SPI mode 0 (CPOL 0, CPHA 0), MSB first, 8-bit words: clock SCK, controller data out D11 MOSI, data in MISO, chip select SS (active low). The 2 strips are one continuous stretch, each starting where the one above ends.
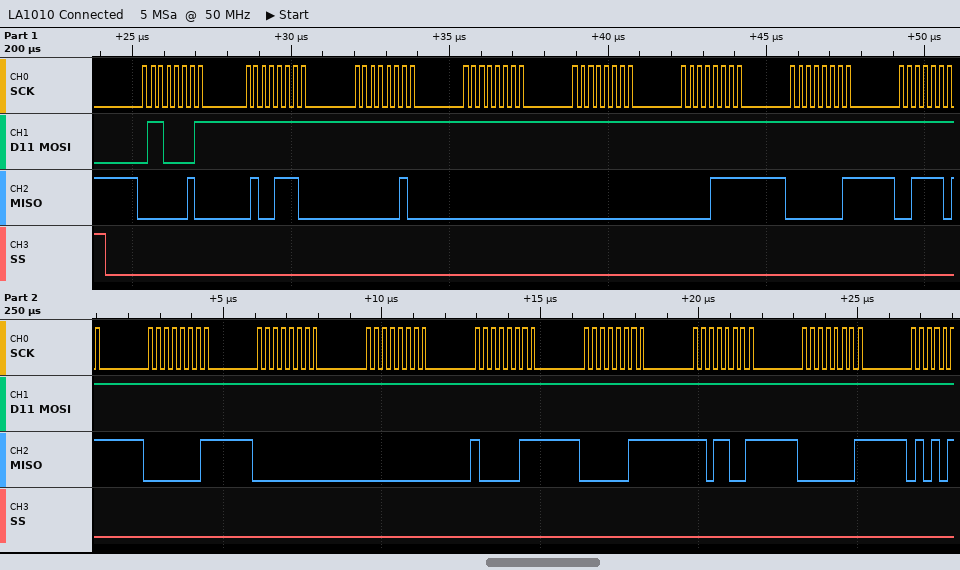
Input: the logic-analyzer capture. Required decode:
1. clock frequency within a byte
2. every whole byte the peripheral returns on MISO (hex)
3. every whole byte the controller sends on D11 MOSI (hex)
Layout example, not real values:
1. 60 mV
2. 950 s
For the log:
1. 4 MHz
2. 0x02 0x4E 0x02 0x00 0x00 0x0F 0x01 0x3D 0x01 0x00 0x00 0x83 0x03 0xD9 0x01
3. 0x61 0xFF 0xFF 0xFF 0xFF 0xFF 0xFF 0xFF 0xFF 0xFF 0xFF 0xFF 0xFF 0xFF 0xFF
